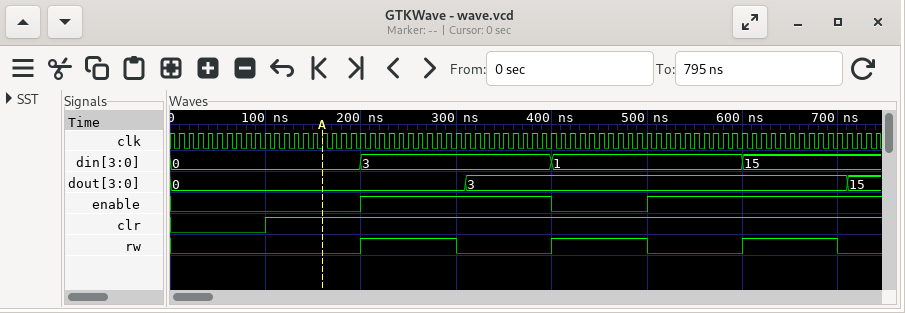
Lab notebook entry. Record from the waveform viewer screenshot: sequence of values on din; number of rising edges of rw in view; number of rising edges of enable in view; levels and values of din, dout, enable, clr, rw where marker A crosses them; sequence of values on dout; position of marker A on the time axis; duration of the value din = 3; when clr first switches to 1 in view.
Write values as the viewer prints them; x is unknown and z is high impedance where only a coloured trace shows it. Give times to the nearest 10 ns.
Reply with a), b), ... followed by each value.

a) 0, 3, 1, 15
b) 3
c) 2
d) din=0, dout=0, enable=0, clr=1, rw=0
e) 0, 3, 15
f) 160 ns
g) 200 ns
h) 100 ns
